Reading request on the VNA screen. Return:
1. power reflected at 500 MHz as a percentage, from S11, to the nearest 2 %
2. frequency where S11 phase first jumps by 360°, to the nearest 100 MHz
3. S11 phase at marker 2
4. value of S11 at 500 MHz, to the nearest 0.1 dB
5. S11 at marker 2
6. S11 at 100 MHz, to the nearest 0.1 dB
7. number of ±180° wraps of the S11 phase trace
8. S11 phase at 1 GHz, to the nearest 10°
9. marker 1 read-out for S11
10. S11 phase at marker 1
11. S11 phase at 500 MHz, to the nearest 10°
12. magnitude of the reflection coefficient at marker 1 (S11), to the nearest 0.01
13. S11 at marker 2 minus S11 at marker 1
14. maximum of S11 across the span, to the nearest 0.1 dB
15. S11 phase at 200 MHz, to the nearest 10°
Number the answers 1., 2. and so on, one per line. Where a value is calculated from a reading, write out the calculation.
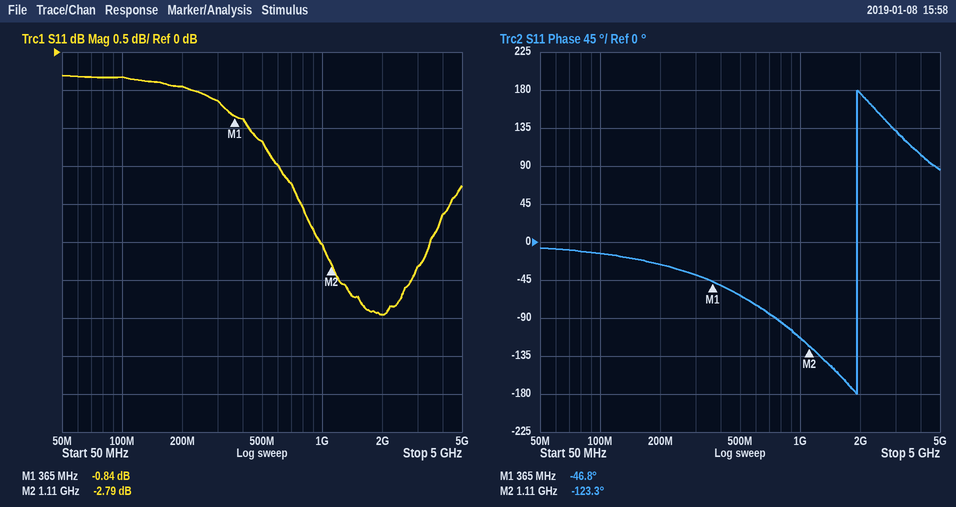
1. 10^(-1.2/10) ≈ 76 %
2. 1.9 GHz
3. -123.3°
4. -1.2 dB
5. -2.79 dB
6. -0.3 dB
7. 1
8. -110°
9. -0.84 dB
10. -46.8°
11. -60°
12. 10^(-0.84/20) ≈ 0.91
13. -2.79 − (-0.84) = -1.95 dB
14. -0.3 dB
15. -30°
